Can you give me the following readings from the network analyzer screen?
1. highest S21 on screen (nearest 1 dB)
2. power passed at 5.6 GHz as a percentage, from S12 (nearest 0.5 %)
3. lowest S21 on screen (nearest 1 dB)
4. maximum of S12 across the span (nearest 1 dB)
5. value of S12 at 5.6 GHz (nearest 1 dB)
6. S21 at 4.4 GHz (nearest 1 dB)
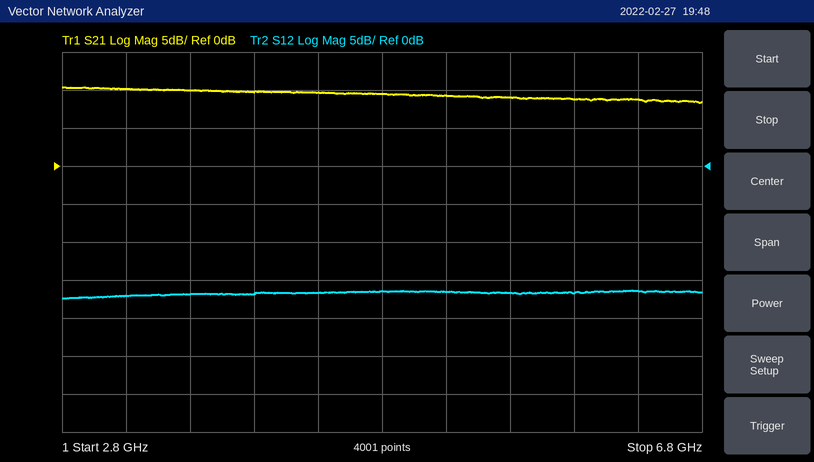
10 dB
2.0 %
8 dB
-16 dB
-17 dB
10 dB
